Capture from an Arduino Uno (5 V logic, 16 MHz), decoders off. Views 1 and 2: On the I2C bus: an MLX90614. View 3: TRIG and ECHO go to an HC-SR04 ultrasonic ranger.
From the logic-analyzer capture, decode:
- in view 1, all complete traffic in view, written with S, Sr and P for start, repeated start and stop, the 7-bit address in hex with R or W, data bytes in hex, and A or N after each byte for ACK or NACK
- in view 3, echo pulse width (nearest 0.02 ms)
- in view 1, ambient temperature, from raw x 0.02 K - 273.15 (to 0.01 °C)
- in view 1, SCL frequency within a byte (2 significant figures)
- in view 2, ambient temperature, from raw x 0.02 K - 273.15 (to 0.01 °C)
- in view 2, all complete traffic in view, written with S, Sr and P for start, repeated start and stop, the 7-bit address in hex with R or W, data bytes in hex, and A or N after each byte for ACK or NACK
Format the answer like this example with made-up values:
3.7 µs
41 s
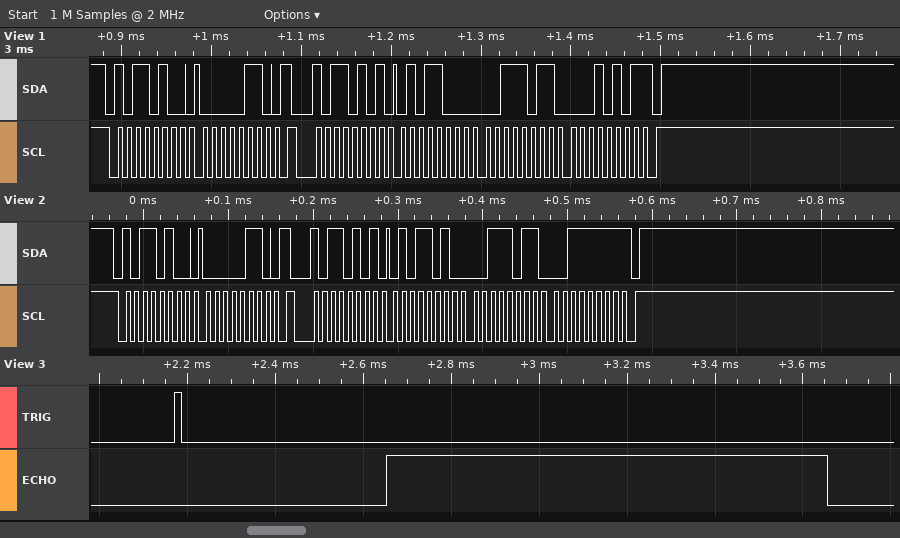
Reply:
S 5AW A 06 A Sr 5AR A 58 A 3B A 15 N P
1.00 ms
30.69 °C
100 kHz
30.73 °C
S 5AW A 06 A Sr 5AR A 5A A 3B A 3F N P
